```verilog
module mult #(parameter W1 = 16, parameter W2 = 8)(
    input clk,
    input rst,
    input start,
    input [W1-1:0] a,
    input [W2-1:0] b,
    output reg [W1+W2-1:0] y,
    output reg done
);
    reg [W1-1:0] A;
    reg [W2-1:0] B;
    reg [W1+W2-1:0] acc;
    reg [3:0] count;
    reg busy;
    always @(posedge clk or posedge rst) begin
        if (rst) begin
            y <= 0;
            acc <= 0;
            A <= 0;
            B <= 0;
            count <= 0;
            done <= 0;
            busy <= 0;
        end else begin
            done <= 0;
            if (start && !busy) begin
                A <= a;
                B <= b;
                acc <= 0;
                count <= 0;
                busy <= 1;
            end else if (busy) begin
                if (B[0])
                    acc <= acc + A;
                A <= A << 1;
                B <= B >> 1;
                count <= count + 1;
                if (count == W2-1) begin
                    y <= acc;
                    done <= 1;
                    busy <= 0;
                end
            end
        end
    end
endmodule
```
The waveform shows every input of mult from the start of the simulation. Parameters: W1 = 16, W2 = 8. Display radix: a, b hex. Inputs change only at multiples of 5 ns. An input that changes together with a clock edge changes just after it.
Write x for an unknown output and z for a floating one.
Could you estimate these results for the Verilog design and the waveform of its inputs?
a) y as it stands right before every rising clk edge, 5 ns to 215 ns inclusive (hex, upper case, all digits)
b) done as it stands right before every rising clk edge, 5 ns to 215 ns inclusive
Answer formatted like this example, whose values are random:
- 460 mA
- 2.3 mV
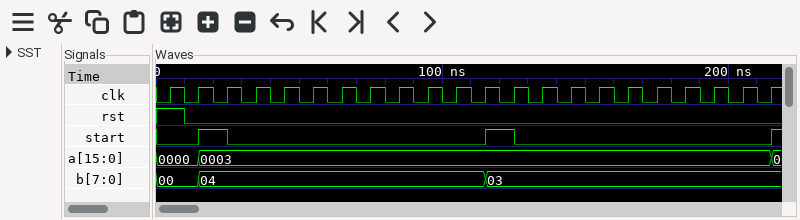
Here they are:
- 000000, 000000, 000000, 000000, 000000, 000000, 000000, 000000, 000000, 000000, 000000, 00000C, 00000C, 00000C, 00000C, 00000C, 00000C, 00000C, 00000C, 00000C, 00000C, 000009
- 0 0 0 0 0 0 0 0 0 0 0 1 0 0 0 0 0 0 0 0 0 1
